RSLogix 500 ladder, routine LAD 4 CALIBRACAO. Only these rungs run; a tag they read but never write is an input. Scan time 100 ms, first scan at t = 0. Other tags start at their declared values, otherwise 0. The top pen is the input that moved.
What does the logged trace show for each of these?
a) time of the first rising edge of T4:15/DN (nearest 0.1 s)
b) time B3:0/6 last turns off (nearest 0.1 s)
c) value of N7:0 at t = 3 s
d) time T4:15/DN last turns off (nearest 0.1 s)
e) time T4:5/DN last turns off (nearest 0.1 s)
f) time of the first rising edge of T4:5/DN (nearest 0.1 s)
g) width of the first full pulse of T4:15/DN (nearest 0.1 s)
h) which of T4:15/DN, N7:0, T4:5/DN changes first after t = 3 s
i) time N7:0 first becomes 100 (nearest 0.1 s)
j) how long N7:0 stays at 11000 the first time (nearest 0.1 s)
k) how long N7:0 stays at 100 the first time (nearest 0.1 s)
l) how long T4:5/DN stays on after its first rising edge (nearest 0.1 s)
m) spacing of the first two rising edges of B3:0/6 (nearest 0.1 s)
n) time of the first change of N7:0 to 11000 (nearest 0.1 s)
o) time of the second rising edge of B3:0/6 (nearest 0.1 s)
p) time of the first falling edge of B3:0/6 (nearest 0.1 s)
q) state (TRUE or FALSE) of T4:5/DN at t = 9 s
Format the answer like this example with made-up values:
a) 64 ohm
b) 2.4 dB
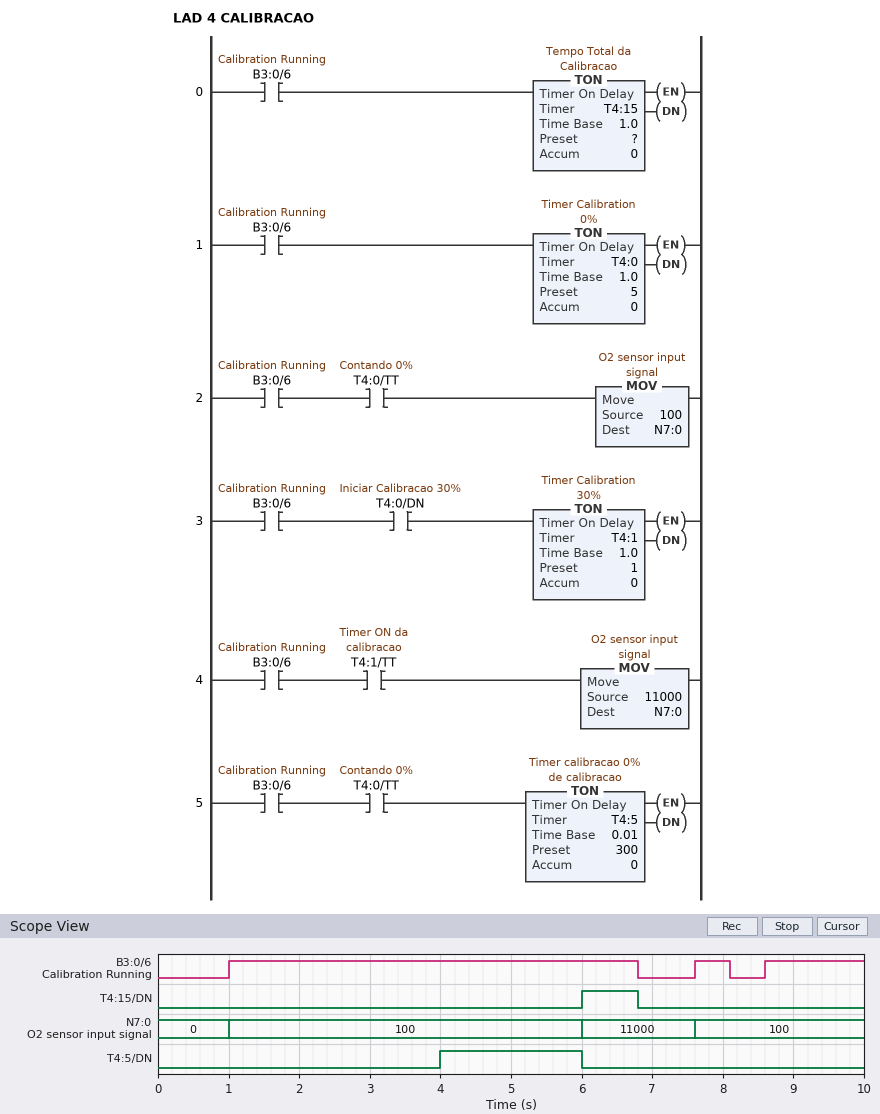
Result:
a) 6.0 s
b) 8.1 s
c) 100
d) 6.8 s
e) 6.0 s
f) 4.0 s
g) 0.8 s
h) T4:5/DN
i) 1.0 s
j) 1.6 s
k) 5.0 s
l) 2.0 s
m) 6.6 s
n) 6.0 s
o) 7.6 s
p) 6.8 s
q) FALSE
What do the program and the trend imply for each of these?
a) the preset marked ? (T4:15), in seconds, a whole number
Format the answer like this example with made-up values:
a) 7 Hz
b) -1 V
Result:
a) 5 s
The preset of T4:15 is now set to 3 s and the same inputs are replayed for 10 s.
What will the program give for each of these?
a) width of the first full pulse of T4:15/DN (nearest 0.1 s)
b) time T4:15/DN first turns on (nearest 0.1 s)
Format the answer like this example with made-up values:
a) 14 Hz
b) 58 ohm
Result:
a) 2.8 s
b) 4.0 s
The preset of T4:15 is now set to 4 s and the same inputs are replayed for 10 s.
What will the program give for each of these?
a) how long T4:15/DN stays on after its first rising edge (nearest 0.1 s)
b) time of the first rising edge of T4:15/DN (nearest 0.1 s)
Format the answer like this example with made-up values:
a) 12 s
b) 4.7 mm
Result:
a) 1.8 s
b) 5.0 s
